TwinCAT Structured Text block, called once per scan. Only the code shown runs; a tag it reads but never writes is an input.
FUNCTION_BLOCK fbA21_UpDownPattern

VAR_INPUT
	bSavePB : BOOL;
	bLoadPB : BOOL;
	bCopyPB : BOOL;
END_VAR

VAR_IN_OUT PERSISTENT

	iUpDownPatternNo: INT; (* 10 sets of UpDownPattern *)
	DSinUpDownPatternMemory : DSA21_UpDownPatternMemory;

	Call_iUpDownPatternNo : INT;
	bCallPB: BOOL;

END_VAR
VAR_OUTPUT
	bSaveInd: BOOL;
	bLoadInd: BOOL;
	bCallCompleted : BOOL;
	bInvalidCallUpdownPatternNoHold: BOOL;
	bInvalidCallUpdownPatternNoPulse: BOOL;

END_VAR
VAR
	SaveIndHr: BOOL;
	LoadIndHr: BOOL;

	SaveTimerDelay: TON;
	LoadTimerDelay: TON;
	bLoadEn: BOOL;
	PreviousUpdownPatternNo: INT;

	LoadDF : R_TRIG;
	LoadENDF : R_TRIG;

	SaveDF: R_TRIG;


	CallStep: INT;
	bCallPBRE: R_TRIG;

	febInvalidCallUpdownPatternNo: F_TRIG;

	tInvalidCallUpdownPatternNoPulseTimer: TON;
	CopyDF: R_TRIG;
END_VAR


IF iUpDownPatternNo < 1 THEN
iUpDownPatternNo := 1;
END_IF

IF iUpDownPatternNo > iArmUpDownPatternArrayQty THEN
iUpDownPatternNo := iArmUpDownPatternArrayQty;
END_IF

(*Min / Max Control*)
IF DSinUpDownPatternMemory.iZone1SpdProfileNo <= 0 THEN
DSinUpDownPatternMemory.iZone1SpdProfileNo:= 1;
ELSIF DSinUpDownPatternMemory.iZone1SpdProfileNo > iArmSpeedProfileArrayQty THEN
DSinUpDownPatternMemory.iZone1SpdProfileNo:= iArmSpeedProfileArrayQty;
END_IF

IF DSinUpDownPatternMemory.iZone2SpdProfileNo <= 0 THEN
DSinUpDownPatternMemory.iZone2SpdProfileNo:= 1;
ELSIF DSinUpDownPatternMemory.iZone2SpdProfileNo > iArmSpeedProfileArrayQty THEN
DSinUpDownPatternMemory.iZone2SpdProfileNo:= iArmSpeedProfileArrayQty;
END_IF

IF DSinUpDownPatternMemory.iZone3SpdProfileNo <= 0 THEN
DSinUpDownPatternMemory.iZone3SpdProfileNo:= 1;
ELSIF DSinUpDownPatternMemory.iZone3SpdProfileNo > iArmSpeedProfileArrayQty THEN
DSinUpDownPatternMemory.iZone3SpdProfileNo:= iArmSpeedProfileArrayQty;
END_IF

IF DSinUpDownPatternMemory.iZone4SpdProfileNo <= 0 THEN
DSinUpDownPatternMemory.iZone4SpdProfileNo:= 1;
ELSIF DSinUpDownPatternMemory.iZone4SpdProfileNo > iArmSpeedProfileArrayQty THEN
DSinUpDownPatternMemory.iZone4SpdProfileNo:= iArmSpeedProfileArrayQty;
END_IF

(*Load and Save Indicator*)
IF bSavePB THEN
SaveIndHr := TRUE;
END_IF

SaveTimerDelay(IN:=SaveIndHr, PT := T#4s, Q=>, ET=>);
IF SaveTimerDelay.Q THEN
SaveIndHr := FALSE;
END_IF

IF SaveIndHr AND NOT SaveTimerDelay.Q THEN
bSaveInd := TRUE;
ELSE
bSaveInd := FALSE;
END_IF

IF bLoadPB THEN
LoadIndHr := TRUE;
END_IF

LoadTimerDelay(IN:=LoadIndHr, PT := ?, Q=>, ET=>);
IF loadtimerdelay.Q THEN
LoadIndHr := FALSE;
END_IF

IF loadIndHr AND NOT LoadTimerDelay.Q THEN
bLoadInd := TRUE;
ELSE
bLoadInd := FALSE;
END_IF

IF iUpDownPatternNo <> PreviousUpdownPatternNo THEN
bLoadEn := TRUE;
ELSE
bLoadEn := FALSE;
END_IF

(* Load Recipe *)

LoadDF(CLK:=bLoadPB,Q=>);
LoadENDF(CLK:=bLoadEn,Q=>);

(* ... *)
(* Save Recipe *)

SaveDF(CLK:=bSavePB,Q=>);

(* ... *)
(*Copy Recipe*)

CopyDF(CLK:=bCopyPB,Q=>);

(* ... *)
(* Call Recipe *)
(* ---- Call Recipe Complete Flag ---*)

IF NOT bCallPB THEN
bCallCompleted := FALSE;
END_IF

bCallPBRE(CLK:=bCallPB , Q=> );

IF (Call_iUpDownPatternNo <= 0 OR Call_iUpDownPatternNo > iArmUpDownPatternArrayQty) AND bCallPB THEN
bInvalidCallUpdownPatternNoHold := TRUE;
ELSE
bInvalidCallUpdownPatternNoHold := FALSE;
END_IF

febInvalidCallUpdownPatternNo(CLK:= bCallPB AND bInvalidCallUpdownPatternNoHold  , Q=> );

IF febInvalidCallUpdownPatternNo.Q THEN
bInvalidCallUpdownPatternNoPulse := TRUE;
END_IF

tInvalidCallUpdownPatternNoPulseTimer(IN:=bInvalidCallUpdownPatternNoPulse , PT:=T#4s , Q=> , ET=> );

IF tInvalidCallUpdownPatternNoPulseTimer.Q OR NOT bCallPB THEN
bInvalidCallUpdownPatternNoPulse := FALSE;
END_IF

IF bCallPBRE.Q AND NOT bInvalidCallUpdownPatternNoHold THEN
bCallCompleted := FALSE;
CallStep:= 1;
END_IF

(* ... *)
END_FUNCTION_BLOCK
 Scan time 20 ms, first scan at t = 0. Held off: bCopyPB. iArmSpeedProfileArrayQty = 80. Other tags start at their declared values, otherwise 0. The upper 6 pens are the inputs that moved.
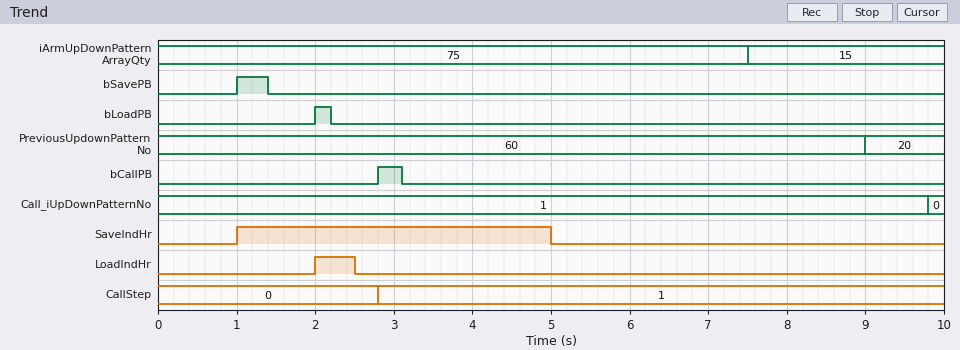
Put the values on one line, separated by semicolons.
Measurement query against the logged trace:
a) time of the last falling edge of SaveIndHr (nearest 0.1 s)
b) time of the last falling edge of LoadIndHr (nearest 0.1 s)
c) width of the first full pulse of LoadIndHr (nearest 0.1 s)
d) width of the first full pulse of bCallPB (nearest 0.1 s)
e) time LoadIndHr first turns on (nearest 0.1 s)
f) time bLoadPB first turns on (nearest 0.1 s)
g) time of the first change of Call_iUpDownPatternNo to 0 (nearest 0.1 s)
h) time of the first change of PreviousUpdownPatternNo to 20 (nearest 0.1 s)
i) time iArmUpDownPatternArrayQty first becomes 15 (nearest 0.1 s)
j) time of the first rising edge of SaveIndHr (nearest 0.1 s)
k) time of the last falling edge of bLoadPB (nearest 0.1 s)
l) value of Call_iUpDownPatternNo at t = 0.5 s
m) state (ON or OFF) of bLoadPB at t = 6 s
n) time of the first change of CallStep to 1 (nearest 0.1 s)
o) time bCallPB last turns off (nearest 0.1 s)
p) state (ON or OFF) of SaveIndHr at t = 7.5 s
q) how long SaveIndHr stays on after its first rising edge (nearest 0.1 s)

5.0 s; 2.5 s; 0.5 s; 0.3 s; 2.0 s; 2.0 s; 9.8 s; 9.0 s; 7.5 s; 1.0 s; 2.2 s; 1; OFF; 2.8 s; 3.1 s; OFF; 4.0 s
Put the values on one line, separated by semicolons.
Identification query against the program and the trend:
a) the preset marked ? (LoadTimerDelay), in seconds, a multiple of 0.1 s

0.5 s
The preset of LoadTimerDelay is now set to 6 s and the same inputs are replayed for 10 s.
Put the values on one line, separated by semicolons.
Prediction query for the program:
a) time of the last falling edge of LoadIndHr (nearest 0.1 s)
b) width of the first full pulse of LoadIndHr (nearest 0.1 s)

8.0 s; 6.0 s
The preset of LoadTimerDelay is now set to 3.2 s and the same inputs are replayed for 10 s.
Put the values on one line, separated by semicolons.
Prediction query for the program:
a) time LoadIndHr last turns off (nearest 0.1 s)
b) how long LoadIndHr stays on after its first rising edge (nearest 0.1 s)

5.2 s; 3.2 s
